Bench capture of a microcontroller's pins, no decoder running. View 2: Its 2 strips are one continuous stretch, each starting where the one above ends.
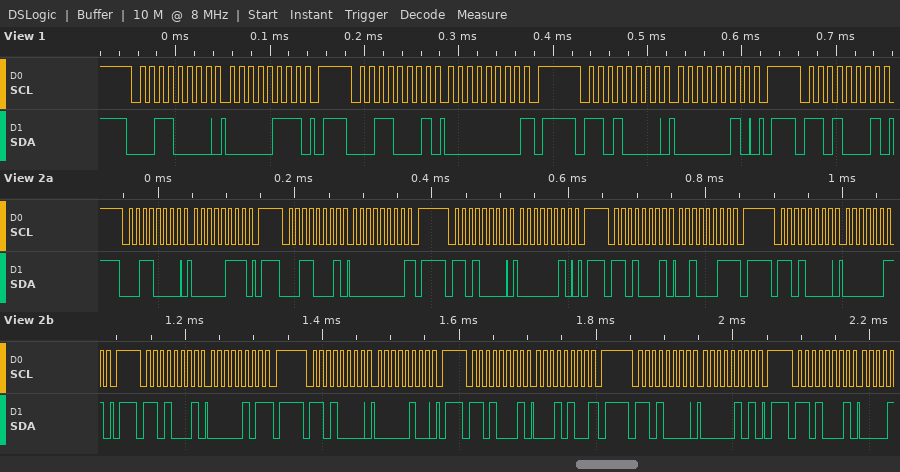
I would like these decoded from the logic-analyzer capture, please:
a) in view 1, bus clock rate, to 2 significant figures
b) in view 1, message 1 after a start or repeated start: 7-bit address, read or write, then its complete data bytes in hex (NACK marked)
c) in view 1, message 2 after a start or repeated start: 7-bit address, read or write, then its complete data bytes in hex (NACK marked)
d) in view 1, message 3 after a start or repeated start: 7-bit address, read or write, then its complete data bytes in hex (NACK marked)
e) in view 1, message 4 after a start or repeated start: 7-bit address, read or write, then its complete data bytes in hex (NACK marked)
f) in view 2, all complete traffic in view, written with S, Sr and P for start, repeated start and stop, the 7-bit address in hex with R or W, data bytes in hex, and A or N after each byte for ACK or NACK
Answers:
100 kHz
0x18 write: 07
0x18 read: 00 NACK
0x68 write: 02
0x68 read
S 18W A 07 A P S 18R A 00 N P S 68W A 02 A P S 68R A 23 N P S 68W A 03 A P S 68R A 05 N P S 68W A 04 A P S 68R A 14 N P S 68W A 05 A P S 68R A
